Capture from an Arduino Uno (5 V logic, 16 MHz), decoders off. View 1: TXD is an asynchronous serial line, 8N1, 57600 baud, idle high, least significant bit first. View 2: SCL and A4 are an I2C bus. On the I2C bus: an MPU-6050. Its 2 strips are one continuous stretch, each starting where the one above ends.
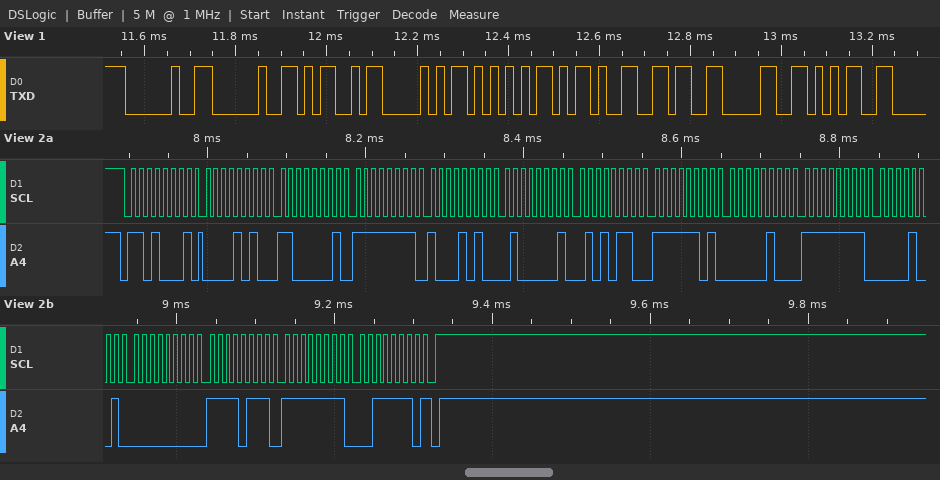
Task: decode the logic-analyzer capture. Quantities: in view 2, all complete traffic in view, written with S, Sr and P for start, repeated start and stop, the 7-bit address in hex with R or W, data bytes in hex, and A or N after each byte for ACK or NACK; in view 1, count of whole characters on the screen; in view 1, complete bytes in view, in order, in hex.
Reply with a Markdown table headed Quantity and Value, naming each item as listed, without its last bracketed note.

| Quantity | Value |
|---|---|
| in view 2, all complete traffic in view, written with S, Sr and P for start, repeated start and stop, the 7-bit address in hex with R or W, data bytes in hex, and A or N after each byte for ACK or NACK | S 68R A 0A A C1 A FF A 8A A 41 A 56 A FD A 04 A FF A 09 A 00 A F7 A FF A 3E N P |
| in view 1, count of whole characters on the screen | 9 |
| in view 1, complete bytes in view, in order, in hex | 20 20 4D 50 55 2D 36 30 35 |
